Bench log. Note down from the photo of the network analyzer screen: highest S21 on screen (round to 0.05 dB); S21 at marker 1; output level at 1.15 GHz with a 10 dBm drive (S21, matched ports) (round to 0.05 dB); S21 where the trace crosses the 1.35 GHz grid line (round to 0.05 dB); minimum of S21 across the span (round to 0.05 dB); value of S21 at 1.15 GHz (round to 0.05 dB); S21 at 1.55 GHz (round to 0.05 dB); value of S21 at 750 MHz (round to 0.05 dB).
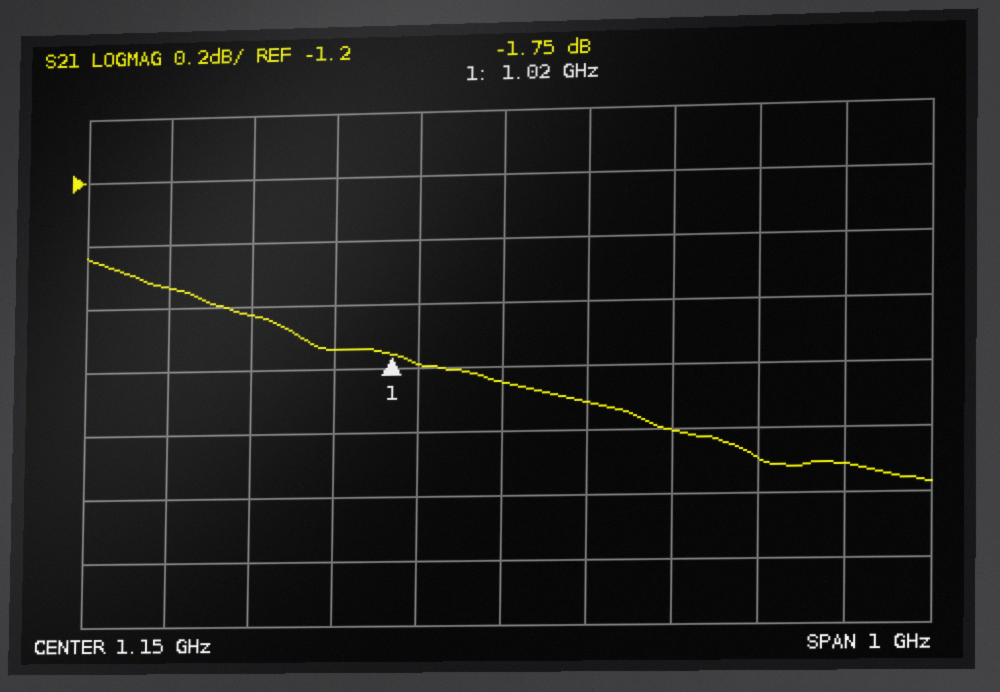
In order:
-1.45 dB
-1.75 dB
8.15 dBm
-2.00 dB
-2.15 dB
-1.85 dB
-2.10 dB
-1.55 dB
